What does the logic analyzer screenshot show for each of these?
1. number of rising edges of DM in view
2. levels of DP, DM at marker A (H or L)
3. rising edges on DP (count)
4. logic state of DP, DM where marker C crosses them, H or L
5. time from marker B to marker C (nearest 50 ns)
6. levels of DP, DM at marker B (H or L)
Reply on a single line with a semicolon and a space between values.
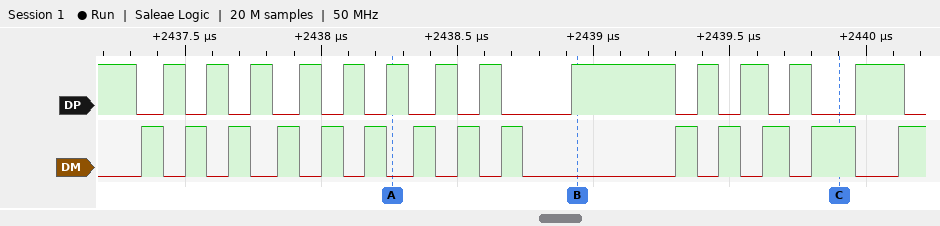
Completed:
14; DP=H, DM=L; 13; DP=L, DM=H; 950 ns; DP=H, DM=L
